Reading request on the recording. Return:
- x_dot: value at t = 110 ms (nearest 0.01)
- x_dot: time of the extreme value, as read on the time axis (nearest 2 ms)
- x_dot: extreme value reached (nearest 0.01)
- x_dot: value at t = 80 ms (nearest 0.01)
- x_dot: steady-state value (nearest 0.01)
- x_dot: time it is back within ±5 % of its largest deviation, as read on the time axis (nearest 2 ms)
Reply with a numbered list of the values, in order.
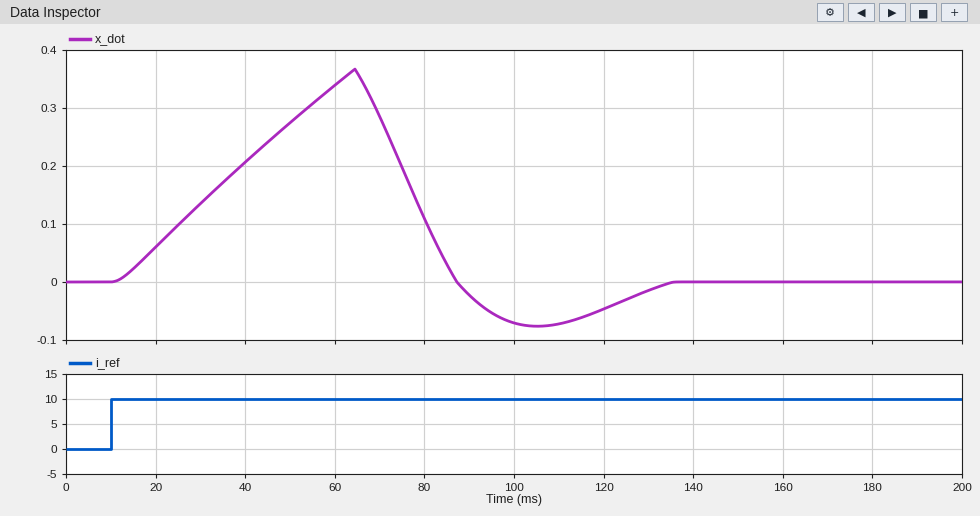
1. -0.07
2. 64 ms
3. 0.37
4. 0.11
5. 0.00
6. 128 ms
